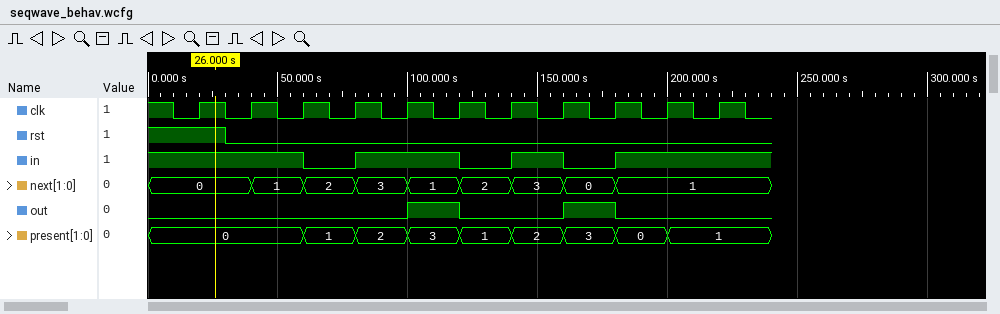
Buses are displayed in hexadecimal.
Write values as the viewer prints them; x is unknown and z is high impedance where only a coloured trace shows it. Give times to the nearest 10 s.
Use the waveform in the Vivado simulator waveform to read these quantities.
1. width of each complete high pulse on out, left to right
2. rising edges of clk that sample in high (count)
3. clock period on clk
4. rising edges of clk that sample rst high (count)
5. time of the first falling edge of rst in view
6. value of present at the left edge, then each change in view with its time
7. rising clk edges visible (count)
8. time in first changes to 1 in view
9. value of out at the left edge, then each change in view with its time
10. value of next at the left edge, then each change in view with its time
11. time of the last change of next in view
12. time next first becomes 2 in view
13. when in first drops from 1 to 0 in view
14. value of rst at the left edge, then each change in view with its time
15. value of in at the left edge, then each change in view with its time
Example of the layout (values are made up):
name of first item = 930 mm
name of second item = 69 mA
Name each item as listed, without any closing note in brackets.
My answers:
width of each complete high pulse on out, left to right = 20 s, 20 s
rising edges of clk that sample in high = 8
clock period on clk = 20 s
rising edges of clk that sample rst high = 1
time of the first falling edge of rst in view = 30 s
value of present at the left edge, then each change in view with its time = 0, 1 at 60 s, 2 at 80 s, 3 at 100 s, 1 at 120 s, 2 at 140 s, 3 at 160 s, 0 at 180 s, 1 at 200 s
rising clk edges visible = 11
time in first changes to 1 in view = 80 s
value of out at the left edge, then each change in view with its time = 0, 1 at 100 s, 0 at 120 s, 1 at 160 s, 0 at 180 s
value of next at the left edge, then each change in view with its time = 0, 1 at 40 s, 2 at 60 s, 3 at 80 s, 1 at 100 s, 2 at 120 s, 3 at 140 s, 0 at 160 s, 1 at 180 s
time of the last change of next in view = 180 s
time next first becomes 2 in view = 60 s
when in first drops from 1 to 0 in view = 60 s
value of rst at the left edge, then each change in view with its time = 1, 0 at 30 s
value of in at the left edge, then each change in view with its time = 1, 0 at 60 s, 1 at 80 s, 0 at 120 s, 1 at 140 s, 0 at 160 s, 1 at 180 s
